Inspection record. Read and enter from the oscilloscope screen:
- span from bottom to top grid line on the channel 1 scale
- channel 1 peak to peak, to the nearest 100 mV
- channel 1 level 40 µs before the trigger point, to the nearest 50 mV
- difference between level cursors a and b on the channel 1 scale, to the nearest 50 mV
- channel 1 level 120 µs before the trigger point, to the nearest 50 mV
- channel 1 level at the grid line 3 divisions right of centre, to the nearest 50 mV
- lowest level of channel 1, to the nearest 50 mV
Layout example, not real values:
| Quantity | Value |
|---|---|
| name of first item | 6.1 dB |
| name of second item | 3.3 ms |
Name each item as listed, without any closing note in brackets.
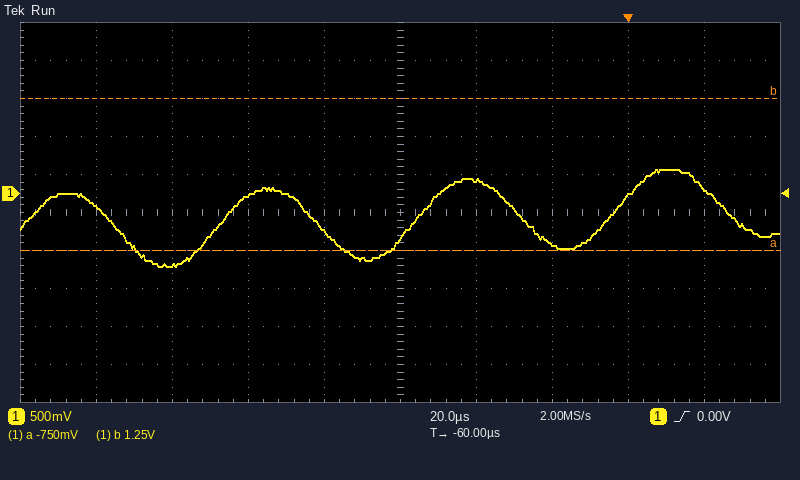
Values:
| Quantity | Value |
|---|---|
| span from bottom to top grid line on the channel 1 scale | 5 V |
| channel 1 peak to peak, to the nearest 100 mV | 1.30 V |
| channel 1 level 40 µs before the trigger point, to the nearest 50 mV | 200 mV |
| difference between level cursors a and b on the channel 1 scale, to the nearest 50 mV | 2.00 V |
| channel 1 level 120 µs before the trigger point, to the nearest 50 mV | -950 mV |
| channel 1 level at the grid line 3 divisions right of centre, to the nearest 50 mV | -50 mV |
| lowest level of channel 1, to the nearest 50 mV | -950 mV |
